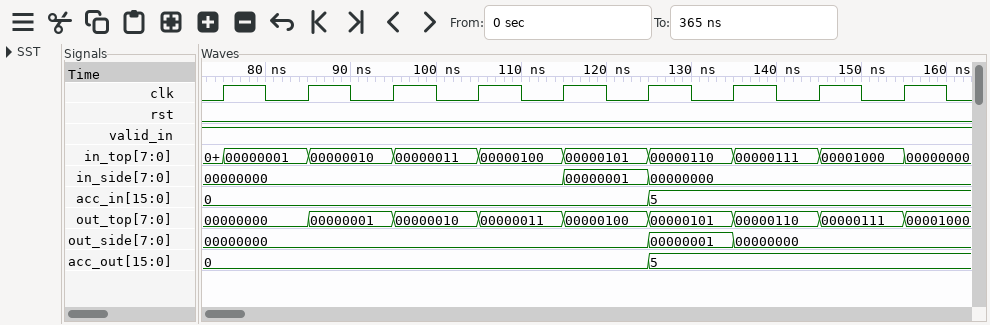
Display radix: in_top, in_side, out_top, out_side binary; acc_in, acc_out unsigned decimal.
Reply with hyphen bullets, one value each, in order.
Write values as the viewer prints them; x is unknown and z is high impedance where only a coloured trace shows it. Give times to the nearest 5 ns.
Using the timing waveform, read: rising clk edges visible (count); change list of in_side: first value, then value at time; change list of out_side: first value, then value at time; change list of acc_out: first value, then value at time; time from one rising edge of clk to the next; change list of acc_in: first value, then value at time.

- 9
- 00000000, 00000001 at 115 ns, 00000000 at 125 ns
- 00000000, 00000001 at 125 ns, 00000000 at 135 ns
- 0, 5 at 125 ns
- 10 ns
- 0, 5 at 125 ns
